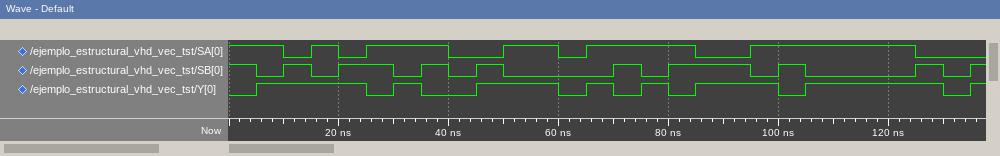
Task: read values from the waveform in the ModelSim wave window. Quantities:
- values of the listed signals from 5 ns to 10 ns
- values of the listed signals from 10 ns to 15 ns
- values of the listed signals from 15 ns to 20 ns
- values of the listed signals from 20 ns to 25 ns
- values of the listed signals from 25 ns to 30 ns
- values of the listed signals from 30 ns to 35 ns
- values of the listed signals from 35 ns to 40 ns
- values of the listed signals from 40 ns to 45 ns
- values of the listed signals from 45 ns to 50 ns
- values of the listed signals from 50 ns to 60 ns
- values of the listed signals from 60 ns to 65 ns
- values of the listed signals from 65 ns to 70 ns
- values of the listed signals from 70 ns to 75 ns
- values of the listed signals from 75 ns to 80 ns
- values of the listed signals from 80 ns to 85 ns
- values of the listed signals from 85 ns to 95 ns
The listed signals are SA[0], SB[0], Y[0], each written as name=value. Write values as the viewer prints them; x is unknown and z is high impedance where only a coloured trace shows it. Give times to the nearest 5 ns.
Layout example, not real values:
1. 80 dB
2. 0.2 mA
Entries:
1. SA[0]=1, SB[0]=0, Y[0]=1
2. SA[0]=0, SB[0]=1, Y[0]=1
3. SA[0]=1, SB[0]=0, Y[0]=1
4. SA[0]=0, SB[0]=1, Y[0]=1
5. SA[0]=1, SB[0]=1, Y[0]=0
6. SA[0]=1, SB[0]=0, Y[0]=1
7. SA[0]=1, SB[0]=1, Y[0]=0
8. SA[0]=0, SB[0]=0, Y[0]=0
9. SA[0]=0, SB[0]=1, Y[0]=1
10. SA[0]=1, SB[0]=0, Y[0]=1
11. SA[0]=0, SB[0]=0, Y[0]=0
12. SA[0]=1, SB[0]=0, Y[0]=1
13. SA[0]=1, SB[0]=1, Y[0]=0
14. SA[0]=1, SB[0]=0, Y[0]=1
15. SA[0]=1, SB[0]=1, Y[0]=0
16. SA[0]=0, SB[0]=1, Y[0]=1
